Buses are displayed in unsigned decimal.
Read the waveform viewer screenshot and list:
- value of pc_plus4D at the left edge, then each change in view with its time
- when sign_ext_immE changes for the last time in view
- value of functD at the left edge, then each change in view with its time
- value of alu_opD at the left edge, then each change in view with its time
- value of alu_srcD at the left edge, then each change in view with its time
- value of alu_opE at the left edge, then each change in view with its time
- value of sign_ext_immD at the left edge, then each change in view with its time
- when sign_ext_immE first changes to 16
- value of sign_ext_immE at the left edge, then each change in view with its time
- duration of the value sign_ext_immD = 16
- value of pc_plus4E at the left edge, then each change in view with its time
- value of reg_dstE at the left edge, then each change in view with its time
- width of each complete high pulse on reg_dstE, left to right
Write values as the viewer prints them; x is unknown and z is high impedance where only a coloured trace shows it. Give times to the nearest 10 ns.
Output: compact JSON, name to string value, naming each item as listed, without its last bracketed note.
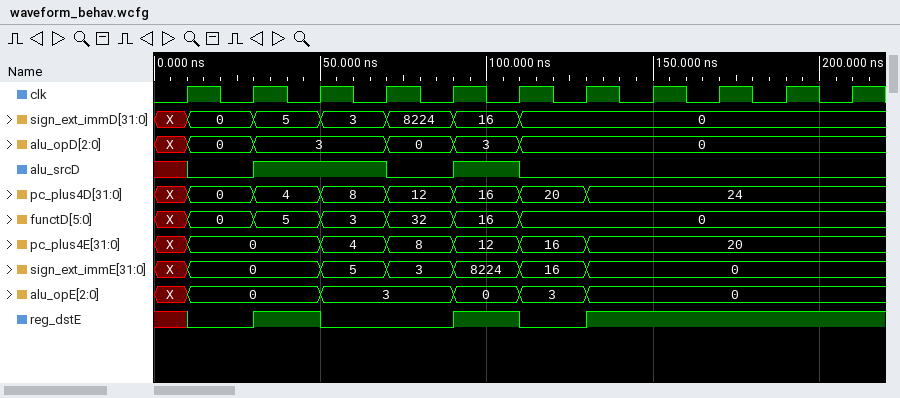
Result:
{"value of pc_plus4D at the left edge, then each change in view with its time": "X, 0 at 10 ns, 4 at 30 ns, 8 at 50 ns, 12 at 70 ns, 16 at 90 ns, 20 at 110 ns, 24 at 130 ns", "when sign_ext_immE changes for the last time in view": "130 ns", "value of functD at the left edge, then each change in view with its time": "X, 0 at 10 ns, 5 at 30 ns, 3 at 50 ns, 32 at 70 ns, 16 at 90 ns, 0 at 110 ns", "value of alu_opD at the left edge, then each change in view with its time": "X, 0 at 10 ns, 3 at 30 ns, 0 at 70 ns, 3 at 90 ns, 0 at 110 ns", "value of alu_srcD at the left edge, then each change in view with its time": "x, 0 at 10 ns, 1 at 30 ns, 0 at 70 ns, 1 at 90 ns, 0 at 110 ns", "value of alu_opE at the left edge, then each change in view with its time": "X, 0 at 10 ns, 3 at 50 ns, 0 at 90 ns, 3 at 110 ns, 0 at 130 ns", "value of sign_ext_immD at the left edge, then each change in view with its time": "X, 0 at 10 ns, 5 at 30 ns, 3 at 50 ns, 8224 at 70 ns, 16 at 90 ns, 0 at 110 ns", "when sign_ext_immE first changes to 16": "110 ns", "value of sign_ext_immE at the left edge, then each change in view with its time": "X, 0 at 10 ns, 5 at 50 ns, 3 at 70 ns, 8224 at 90 ns, 16 at 110 ns, 0 at 130 ns", "duration of the value sign_ext_immD = 16": "20 ns", "value of pc_plus4E at the left edge, then each change in view with its time": "X, 0 at 10 ns, 4 at 50 ns, 8 at 70 ns, 12 at 90 ns, 16 at 110 ns, 20 at 130 ns", "value of reg_dstE at the left edge, then each change in view with its time": "x, 0 at 10 ns, 1 at 30 ns, 0 at 50 ns, 1 at 90 ns, 0 at 110 ns, 1 at 130 ns", "width of each complete high pulse on reg_dstE, left to right": "20 ns, 20 ns"}
